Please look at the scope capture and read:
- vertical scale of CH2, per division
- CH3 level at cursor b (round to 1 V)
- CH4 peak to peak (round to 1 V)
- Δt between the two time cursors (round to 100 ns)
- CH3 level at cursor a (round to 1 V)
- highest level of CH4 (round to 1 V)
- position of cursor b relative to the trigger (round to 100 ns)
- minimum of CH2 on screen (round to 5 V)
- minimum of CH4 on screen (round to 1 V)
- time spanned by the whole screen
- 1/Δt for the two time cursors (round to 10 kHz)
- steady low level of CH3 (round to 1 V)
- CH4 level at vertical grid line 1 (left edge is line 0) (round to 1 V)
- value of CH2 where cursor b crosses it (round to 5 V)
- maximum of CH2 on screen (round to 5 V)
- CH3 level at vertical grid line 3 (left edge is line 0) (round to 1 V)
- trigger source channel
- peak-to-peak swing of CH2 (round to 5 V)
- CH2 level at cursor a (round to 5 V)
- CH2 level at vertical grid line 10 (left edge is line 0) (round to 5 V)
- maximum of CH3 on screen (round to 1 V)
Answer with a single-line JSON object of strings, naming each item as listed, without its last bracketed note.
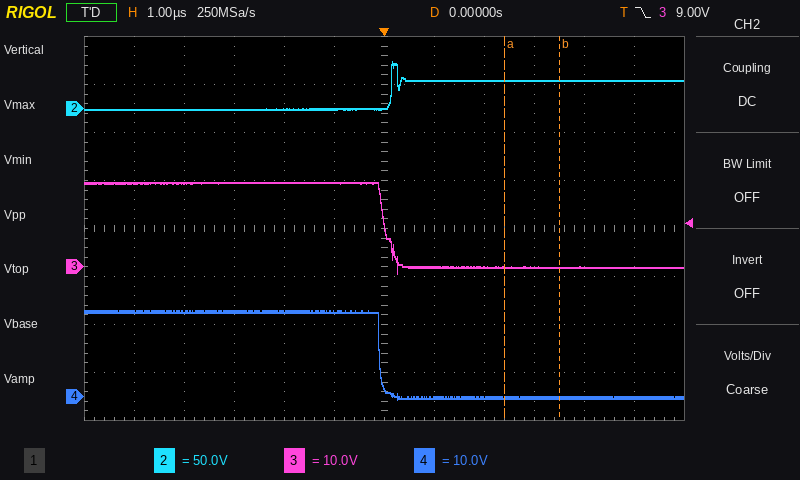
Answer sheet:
{"vertical scale of CH2, per division": "50 V", "CH3 level at cursor b": "0 V", "CH4 peak to peak": "19 V", "Δt between the two time cursors": "1.1 µs", "CH3 level at cursor a": "0 V", "highest level of CH4": "18 V", "position of cursor b relative to the trigger": "+3.5 µs", "minimum of CH2 on screen": "0 V", "minimum of CH4 on screen": "-1 V", "time spanned by the whole screen": "12 µs", "1/Δt for the two time cursors": "910 kHz", "steady low level of CH3": "0 V", "CH4 level at vertical grid line 1 (left edge is line 0)": "18 V", "value of CH2 where cursor b crosses it": "30 V", "maximum of CH2 on screen": "50 V", "CH3 level at vertical grid line 3 (left edge is line 0)": "18 V", "trigger source channel": "CH3", "peak-to-peak swing of CH2": "50 V", "CH2 level at cursor a": "30 V", "CH2 level at vertical grid line 10 (left edge is line 0)": "30 V", "maximum of CH3 on screen": "18 V"}
